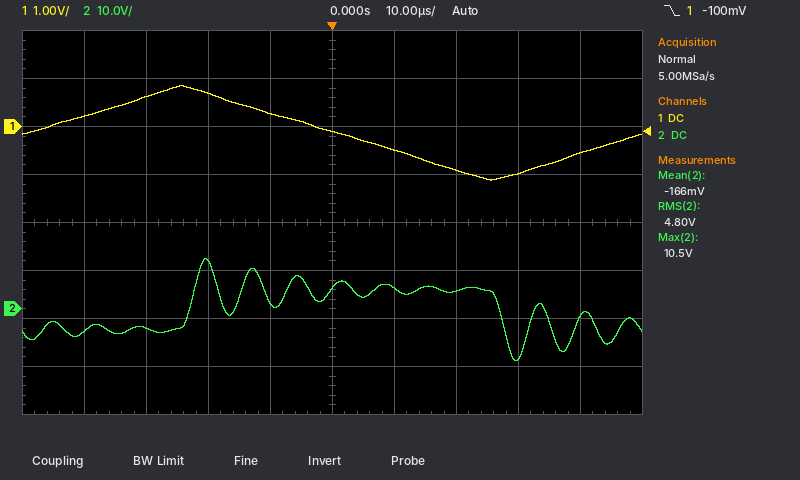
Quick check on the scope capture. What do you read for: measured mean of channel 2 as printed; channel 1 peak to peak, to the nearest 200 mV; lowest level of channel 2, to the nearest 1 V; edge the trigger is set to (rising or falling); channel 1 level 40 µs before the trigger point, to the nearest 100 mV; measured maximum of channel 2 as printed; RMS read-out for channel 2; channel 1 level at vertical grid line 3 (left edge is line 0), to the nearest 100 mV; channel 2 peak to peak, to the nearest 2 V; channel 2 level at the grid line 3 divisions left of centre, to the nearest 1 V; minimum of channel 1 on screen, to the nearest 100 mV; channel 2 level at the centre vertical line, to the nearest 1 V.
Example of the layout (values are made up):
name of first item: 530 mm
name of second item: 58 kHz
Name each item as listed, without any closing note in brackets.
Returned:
measured mean of channel 2 as printed: -166 mV
channel 1 peak to peak, to the nearest 200 mV: 2.0 V
lowest level of channel 2, to the nearest 1 V: -11 V
edge the trigger is set to: falling
channel 1 level 40 µs before the trigger point, to the nearest 100 mV: 200 mV
measured maximum of channel 2 as printed: 10.5 V
RMS read-out for channel 2: 4.80 V
channel 1 level at vertical grid line 3 (left edge is line 0), to the nearest 100 mV: 700 mV
channel 2 peak to peak, to the nearest 2 V: 22 V
channel 2 level at the grid line 3 divisions left of centre, to the nearest 1 V: -4 V
minimum of channel 1 on screen, to the nearest 100 mV: -1.1 V
channel 2 level at the centre vertical line, to the nearest 1 V: 4 V
